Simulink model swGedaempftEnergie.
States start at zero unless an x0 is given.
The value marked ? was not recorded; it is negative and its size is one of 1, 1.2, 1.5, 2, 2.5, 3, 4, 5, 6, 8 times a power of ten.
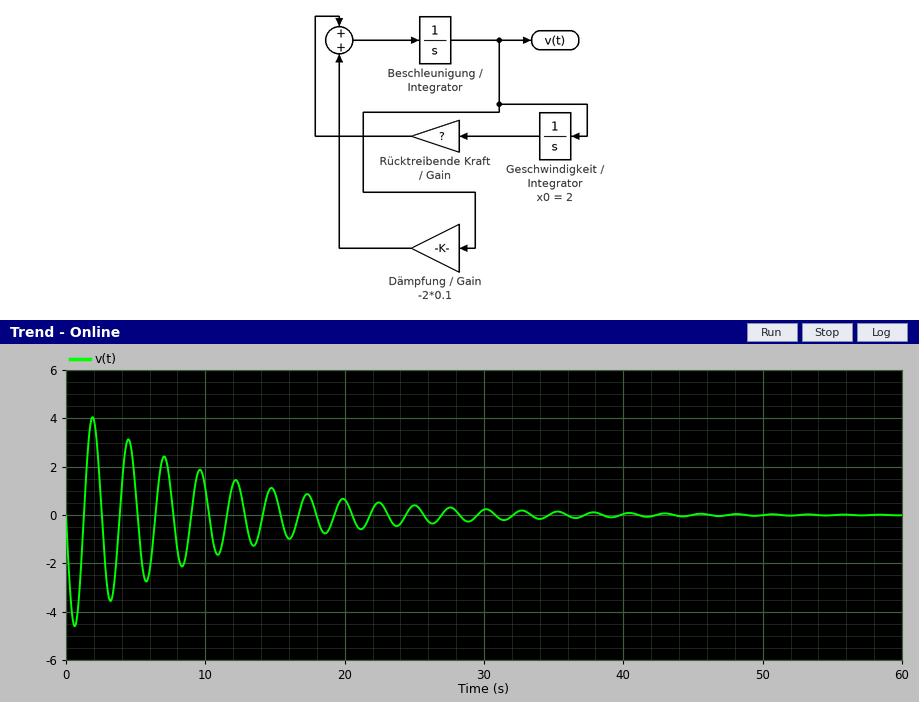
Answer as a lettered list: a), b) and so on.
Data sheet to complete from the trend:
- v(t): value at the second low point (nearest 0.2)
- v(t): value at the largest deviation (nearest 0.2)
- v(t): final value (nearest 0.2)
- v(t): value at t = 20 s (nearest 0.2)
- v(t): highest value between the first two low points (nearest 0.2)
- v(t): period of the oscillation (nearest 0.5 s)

a) -3.6
b) -4.6
c) 0.0
d) 0.6
e) 4.0
f) 2.5 s
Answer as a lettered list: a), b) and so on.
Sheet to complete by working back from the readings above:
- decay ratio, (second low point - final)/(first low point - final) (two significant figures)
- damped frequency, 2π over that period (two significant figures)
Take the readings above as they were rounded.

a) 0.78
b) 2.5 rad/s
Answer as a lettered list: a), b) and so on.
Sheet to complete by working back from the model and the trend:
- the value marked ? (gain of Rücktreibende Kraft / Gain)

a) -6
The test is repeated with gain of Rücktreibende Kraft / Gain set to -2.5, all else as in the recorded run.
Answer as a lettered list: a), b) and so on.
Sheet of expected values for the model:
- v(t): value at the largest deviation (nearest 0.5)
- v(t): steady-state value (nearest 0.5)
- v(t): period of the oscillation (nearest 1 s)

a) -3.0
b) 0.0
c) 4 s
